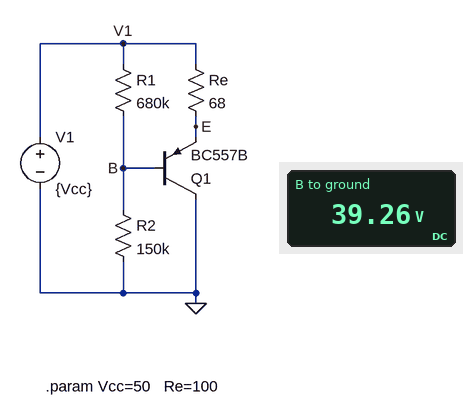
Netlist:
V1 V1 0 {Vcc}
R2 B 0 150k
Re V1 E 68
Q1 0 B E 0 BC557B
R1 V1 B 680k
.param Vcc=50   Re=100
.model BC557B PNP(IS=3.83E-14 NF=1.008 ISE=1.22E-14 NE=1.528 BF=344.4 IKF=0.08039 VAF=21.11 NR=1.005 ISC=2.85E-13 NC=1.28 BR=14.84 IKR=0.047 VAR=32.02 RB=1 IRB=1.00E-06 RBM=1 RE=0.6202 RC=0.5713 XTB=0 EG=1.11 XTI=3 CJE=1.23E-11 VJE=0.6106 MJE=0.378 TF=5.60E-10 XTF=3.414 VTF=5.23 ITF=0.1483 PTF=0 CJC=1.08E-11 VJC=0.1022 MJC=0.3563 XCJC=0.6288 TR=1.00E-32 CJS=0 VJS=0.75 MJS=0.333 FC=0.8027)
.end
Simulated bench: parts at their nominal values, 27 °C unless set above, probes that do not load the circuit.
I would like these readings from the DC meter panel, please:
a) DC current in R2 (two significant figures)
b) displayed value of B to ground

260 µA
39.26 V
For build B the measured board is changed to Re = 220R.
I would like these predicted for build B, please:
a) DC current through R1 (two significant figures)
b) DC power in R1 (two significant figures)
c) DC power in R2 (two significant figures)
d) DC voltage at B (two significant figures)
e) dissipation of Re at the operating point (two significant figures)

30 µA
630 µW
5.7 mW
29 V
1.8 W
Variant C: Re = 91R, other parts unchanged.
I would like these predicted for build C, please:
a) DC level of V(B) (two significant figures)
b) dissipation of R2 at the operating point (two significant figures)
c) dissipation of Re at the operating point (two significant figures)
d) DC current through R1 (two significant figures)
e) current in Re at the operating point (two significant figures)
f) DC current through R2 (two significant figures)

37 V
9.2 mW
1.6 W
19 µA
130 mA
250 µA
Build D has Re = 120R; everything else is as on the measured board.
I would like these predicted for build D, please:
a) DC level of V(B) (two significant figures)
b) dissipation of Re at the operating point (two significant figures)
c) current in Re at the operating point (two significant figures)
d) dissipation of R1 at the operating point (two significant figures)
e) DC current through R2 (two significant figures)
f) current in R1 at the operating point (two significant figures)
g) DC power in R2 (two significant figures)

35 V
1.7 W
120 mA
340 µW
230 µA
22 µA
8.1 mW
